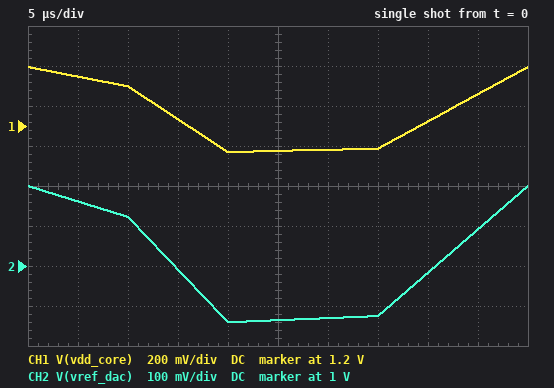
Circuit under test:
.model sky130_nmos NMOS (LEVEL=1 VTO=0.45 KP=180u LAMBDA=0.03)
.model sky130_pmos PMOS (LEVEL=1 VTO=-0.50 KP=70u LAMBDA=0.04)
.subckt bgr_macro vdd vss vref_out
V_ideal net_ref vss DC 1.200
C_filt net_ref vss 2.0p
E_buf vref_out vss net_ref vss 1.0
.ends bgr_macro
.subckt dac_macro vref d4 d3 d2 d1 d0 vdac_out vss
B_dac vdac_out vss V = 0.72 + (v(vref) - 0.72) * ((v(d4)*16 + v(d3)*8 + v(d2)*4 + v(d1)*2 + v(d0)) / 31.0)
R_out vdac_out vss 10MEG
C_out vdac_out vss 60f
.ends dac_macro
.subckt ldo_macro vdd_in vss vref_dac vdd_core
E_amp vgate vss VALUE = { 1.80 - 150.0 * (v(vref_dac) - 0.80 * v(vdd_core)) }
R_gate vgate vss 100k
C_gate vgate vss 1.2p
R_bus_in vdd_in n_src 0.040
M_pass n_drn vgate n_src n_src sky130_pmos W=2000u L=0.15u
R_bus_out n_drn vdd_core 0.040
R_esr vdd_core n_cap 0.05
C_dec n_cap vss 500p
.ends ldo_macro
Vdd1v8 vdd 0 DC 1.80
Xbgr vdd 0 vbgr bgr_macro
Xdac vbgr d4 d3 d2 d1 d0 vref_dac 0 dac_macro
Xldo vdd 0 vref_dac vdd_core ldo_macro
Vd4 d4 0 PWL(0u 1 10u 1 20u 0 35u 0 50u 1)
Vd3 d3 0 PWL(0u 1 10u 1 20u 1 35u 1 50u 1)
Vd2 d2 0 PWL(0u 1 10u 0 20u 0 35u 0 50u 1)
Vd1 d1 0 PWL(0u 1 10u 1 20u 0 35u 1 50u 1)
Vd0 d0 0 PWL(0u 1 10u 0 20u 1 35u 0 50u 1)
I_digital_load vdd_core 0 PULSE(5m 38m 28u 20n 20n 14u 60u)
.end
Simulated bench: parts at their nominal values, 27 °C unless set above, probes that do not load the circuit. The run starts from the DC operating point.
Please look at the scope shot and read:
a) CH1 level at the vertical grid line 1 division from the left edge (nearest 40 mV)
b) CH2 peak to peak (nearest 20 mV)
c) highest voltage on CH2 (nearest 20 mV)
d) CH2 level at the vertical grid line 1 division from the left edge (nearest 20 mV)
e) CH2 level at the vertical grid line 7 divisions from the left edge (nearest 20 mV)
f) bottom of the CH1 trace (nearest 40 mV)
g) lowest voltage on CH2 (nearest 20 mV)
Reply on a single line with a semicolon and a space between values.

1.44 V; 340 mV; 1.20 V; 1.16 V; 880 mV; 1.08 V; 860 mV
